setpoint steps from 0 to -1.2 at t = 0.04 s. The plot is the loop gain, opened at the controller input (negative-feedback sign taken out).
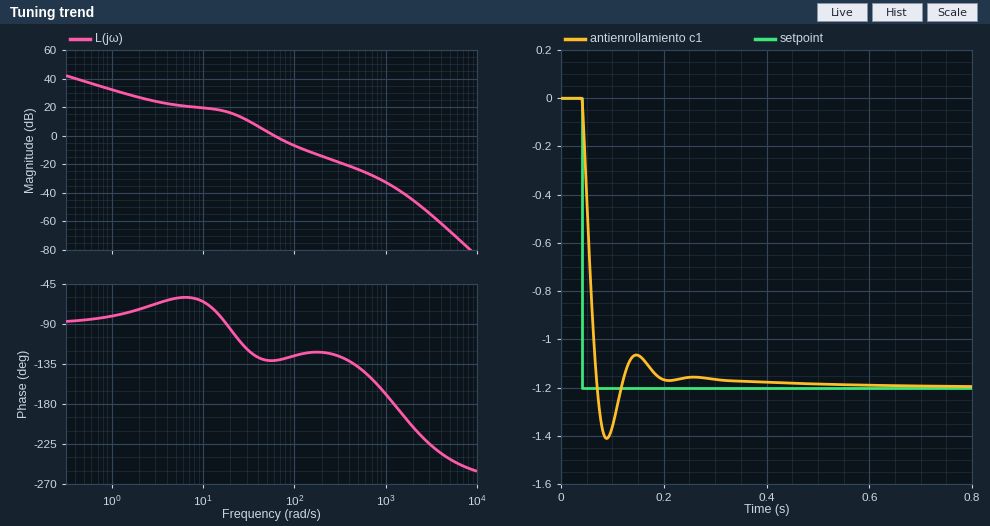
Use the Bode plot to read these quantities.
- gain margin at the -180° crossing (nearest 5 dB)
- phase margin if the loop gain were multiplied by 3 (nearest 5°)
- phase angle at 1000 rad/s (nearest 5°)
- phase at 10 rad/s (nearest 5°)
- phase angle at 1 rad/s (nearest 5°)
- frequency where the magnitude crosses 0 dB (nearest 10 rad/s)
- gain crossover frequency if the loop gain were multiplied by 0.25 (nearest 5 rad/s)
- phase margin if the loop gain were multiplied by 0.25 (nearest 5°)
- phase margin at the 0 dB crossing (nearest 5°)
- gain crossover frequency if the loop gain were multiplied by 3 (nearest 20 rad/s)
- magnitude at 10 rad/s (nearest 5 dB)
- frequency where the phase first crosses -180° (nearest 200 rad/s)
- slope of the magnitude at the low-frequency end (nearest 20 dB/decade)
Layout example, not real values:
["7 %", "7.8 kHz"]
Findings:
["35 dB", "55°", "-170°", "-65°", "-80°", "60 rad/s", "30 rad/s", "65°", "50°", "120 rad/s", "20 dB", "1200 rad/s", "-20 dB/decade"]
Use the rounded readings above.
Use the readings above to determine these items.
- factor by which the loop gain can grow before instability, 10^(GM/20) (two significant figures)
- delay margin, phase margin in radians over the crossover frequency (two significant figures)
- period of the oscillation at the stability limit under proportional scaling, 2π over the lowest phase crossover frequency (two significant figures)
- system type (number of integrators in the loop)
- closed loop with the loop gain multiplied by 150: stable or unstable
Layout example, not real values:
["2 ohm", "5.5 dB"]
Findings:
["56", "0.015 s", "0.0052 s", "1", "unstable"]
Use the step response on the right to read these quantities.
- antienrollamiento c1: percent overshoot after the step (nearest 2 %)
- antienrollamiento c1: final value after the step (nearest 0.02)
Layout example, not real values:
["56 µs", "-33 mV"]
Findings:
["18 %", "-1.20"]
